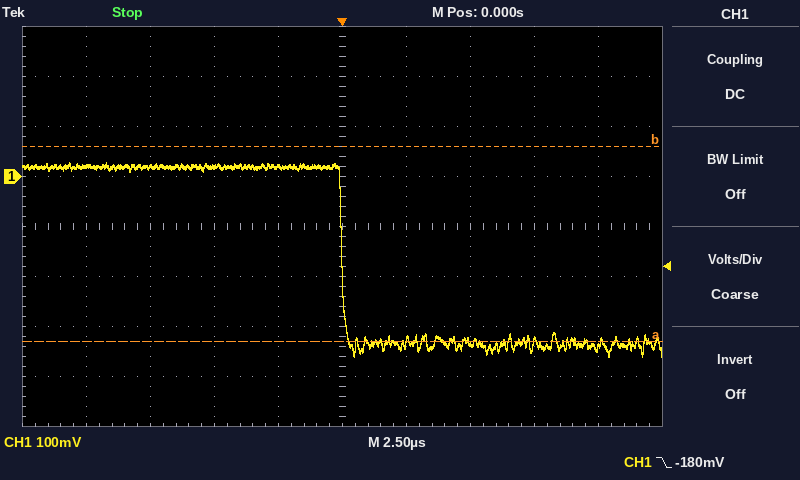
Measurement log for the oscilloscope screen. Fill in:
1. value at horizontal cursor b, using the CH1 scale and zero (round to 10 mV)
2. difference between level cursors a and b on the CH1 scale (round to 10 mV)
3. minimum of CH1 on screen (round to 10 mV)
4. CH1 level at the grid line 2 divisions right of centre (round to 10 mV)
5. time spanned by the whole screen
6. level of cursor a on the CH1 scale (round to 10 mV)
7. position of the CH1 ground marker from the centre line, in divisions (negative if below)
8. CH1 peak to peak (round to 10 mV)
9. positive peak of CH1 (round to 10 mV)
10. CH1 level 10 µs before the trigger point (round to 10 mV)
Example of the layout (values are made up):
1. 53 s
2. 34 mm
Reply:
1. 60 mV
2. 390 mV
3. -360 mV
4. -330 mV
5. 25 µs
6. -330 mV
7. +1.0 div
8. 390 mV
9. 30 mV
10. 20 mV
